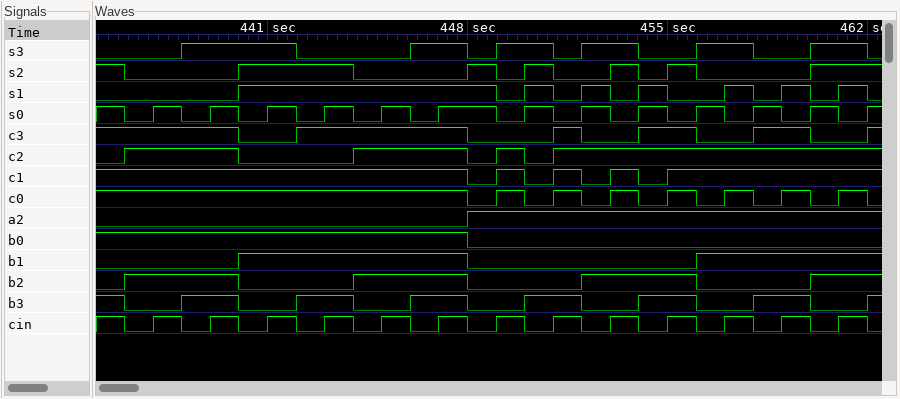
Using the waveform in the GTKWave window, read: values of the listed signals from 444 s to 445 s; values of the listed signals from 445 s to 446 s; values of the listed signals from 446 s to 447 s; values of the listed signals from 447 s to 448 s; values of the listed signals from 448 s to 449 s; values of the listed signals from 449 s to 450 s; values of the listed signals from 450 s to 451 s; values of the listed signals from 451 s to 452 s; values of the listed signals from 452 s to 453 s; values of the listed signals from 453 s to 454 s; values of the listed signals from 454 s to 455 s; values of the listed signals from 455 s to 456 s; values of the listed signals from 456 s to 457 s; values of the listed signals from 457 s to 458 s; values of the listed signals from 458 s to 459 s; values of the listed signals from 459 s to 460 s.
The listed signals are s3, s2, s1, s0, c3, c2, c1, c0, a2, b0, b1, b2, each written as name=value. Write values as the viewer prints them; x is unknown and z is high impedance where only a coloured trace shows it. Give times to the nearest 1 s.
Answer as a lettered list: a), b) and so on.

a) s3=0, s2=0, s1=1, s0=0, c3=1, c2=1, c1=1, c0=1, a2=0, b0=1, b1=1, b2=1
b) s3=0, s2=0, s1=1, s0=1, c3=1, c2=1, c1=1, c0=1, a2=0, b0=1, b1=1, b2=1
c) s3=1, s2=0, s1=1, s0=0, c3=1, c2=1, c1=1, c0=1, a2=0, b0=1, b1=1, b2=1
d) s3=1, s2=0, s1=1, s0=1, c3=1, c2=1, c1=1, c0=1, a2=0, b0=1, b1=1, b2=1
e) s3=0, s2=1, s1=1, s0=1, c3=0, c2=0, c1=0, c0=0, a2=1, b0=0, b1=0, b2=0
f) s3=1, s2=0, s1=0, s0=0, c3=0, c2=1, c1=1, c0=1, a2=1, b0=0, b1=0, b2=0
g) s3=1, s2=1, s1=1, s0=1, c3=0, c2=0, c1=0, c0=0, a2=1, b0=0, b1=0, b2=0
h) s3=0, s2=0, s1=0, s0=0, c3=1, c2=1, c1=1, c0=1, a2=1, b0=0, b1=0, b2=0
i) s3=1, s2=0, s1=1, s0=1, c3=0, c2=1, c1=0, c0=0, a2=1, b0=0, b1=0, b2=1
j) s3=1, s2=1, s1=0, s0=0, c3=0, c2=1, c1=1, c0=1, a2=1, b0=0, b1=0, b2=1
k) s3=0, s2=0, s1=1, s0=1, c3=1, c2=1, c1=0, c0=0, a2=1, b0=0, b1=0, b2=1
l) s3=0, s2=1, s1=0, s0=0, c3=1, c2=1, c1=1, c0=1, a2=1, b0=0, b1=0, b2=1
m) s3=1, s2=0, s1=0, s0=1, c3=0, c2=1, c1=1, c0=0, a2=1, b0=0, b1=1, b2=0
n) s3=1, s2=0, s1=1, s0=0, c3=0, c2=1, c1=1, c0=1, a2=1, b0=0, b1=1, b2=0
o) s3=0, s2=0, s1=0, s0=1, c3=1, c2=1, c1=1, c0=0, a2=1, b0=0, b1=1, b2=0
p) s3=0, s2=0, s1=1, s0=0, c3=1, c2=1, c1=1, c0=1, a2=1, b0=0, b1=1, b2=0
